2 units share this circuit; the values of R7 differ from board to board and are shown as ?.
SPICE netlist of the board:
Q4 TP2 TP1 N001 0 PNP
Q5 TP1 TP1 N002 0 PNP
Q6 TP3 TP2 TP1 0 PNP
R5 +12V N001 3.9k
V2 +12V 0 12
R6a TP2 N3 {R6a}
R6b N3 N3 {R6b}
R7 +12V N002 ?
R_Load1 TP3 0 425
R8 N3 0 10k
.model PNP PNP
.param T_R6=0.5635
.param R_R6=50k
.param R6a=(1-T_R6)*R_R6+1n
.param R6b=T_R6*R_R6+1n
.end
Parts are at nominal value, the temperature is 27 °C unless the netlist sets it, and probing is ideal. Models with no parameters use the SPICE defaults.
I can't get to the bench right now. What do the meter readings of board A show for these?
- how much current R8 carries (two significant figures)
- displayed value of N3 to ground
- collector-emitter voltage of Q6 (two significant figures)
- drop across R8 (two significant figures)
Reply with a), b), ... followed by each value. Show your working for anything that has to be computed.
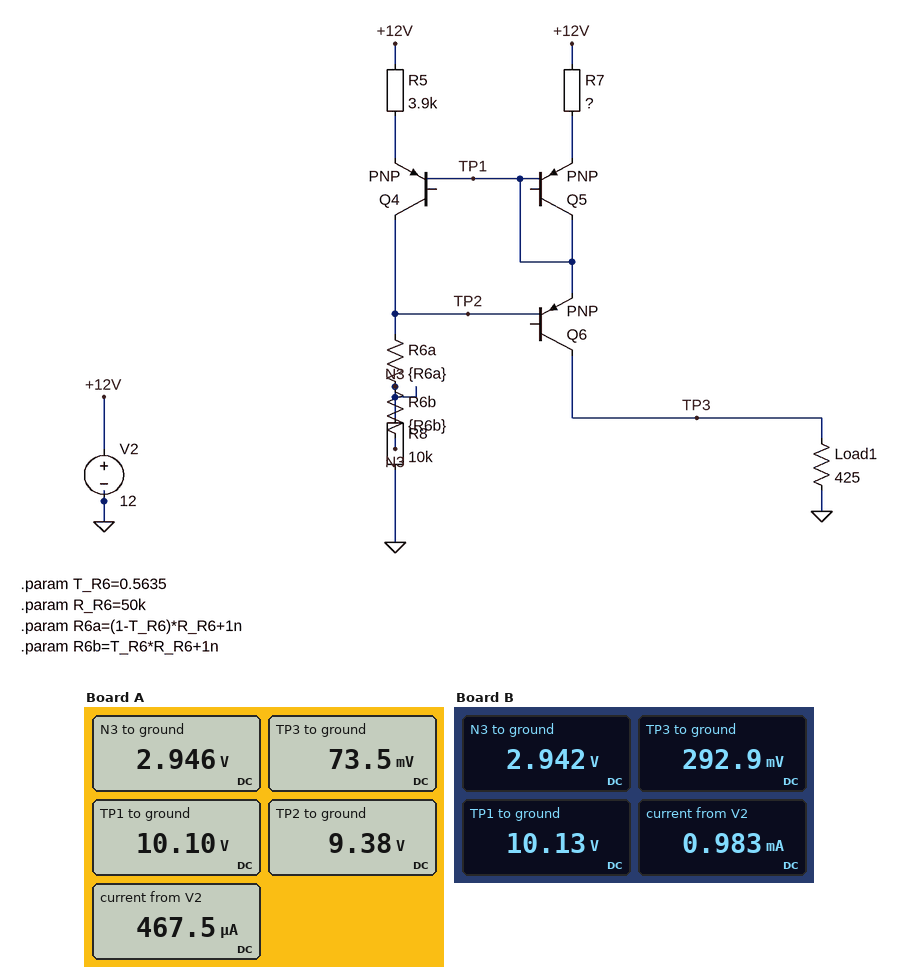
a) (2.946 V) / 10 kΩ = 290 µA
b) 2.946 V
c) 73.5 mV - 10.1 V = -10 V
d) 2.946 V = 2.9 V
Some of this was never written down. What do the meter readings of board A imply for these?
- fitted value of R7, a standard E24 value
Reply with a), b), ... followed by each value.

a) 6.8 kΩ
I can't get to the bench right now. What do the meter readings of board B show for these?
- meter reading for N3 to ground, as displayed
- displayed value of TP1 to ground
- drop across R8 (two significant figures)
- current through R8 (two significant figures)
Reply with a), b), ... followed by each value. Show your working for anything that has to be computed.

a) 2.942 V
b) 10.13 V
c) 2.942 V = 2.9 V
d) (2.942 V) / 10 kΩ = 290 µA
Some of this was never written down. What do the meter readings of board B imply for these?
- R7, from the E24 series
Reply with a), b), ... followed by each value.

a) 1.6 kΩ
